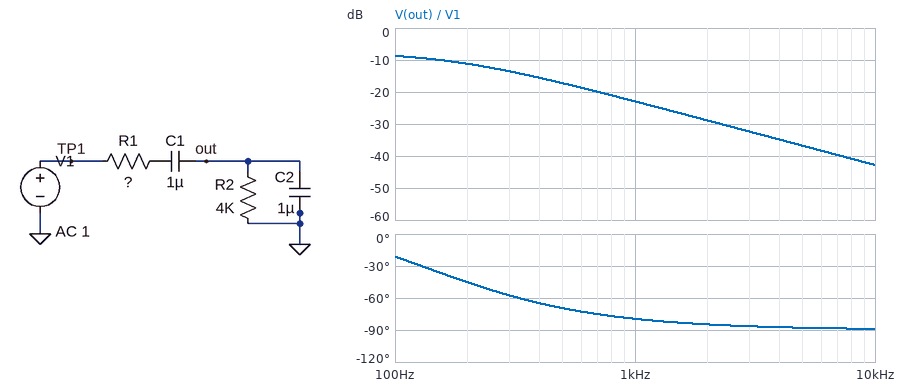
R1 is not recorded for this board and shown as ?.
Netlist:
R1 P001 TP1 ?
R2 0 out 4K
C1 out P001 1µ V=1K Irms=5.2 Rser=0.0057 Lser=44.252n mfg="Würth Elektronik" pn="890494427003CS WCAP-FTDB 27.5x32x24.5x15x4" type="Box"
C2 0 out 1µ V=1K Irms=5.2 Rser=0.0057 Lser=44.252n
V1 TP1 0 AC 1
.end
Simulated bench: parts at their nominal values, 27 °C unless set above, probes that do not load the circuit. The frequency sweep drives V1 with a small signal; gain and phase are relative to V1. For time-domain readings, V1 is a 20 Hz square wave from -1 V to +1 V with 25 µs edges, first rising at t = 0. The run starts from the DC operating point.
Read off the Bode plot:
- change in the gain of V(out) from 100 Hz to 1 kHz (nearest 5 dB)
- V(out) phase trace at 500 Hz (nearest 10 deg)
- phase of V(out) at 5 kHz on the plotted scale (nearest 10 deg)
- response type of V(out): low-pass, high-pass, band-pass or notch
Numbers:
-15 dB
-70 deg
-90 deg
low-pass
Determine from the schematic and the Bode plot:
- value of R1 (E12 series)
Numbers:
2.2 kΩ
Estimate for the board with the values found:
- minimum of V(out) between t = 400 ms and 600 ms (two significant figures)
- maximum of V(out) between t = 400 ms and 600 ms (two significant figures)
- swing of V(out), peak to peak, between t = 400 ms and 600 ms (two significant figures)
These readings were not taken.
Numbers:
-620 mV
620 mV
1.2 V
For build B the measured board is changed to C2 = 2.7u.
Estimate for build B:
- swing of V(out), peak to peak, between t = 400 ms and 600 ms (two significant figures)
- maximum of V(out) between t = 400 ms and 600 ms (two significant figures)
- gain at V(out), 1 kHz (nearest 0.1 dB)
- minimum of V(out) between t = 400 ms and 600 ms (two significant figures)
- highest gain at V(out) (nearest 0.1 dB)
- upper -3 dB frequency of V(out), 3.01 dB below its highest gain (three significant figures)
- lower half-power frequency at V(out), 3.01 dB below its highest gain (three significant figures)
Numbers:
660 mV
330 mV
-31.5 dB
-330 mV
-12.6 dB
123 Hz
8.70 Hz
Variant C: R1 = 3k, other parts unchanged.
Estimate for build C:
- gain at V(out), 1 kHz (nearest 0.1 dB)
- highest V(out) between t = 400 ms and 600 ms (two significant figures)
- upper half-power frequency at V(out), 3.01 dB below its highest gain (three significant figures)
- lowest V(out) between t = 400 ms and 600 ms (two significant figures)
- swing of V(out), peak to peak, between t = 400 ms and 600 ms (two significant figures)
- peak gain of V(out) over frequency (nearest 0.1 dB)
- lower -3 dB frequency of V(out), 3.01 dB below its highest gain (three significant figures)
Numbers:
-25.6 dB
560 mV
159 Hz
-560 mV
1.1 V
-8.8 dB
13.3 Hz
